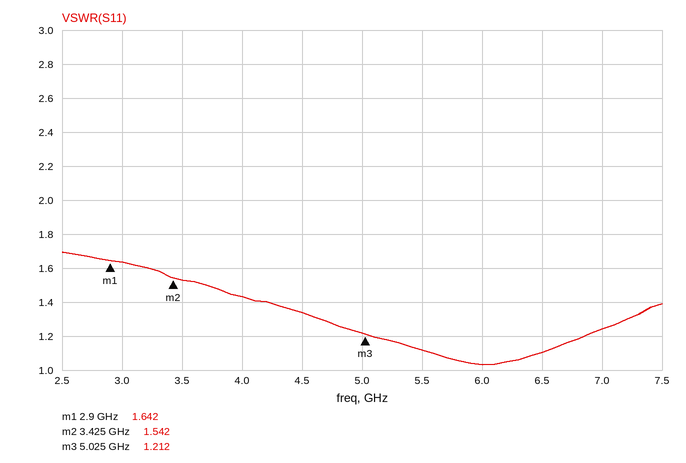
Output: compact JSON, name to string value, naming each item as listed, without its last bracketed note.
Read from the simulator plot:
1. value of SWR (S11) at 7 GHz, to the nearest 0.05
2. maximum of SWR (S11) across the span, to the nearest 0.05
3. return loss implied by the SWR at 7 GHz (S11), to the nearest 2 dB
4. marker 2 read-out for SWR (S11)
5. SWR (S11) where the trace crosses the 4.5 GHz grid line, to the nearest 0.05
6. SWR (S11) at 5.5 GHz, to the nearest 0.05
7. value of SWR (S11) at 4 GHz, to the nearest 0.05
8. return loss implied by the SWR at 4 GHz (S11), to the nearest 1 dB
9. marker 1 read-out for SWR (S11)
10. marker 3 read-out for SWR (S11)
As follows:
{"value of SWR (S11) at 7 GHz, to the nearest 0.05": "1.25", "maximum of SWR (S11) across the span, to the nearest 0.05": "1.70", "return loss implied by the SWR at 7 GHz (S11), to the nearest 2 dB": "20 dB", "marker 2 read-out for SWR": "1.542", "SWR (S11) where the trace crosses the 4.5 GHz grid line, to the nearest 0.05": "1.35", "SWR (S11) at 5.5 GHz, to the nearest 0.05": "1.10", "value of SWR (S11) at 4 GHz, to the nearest 0.05": "1.45", "return loss implied by the SWR at 4 GHz (S11), to the nearest 1 dB": "15 dB", "marker 1 read-out for SWR": "1.642", "marker 3 read-out for SWR": "1.212"}
